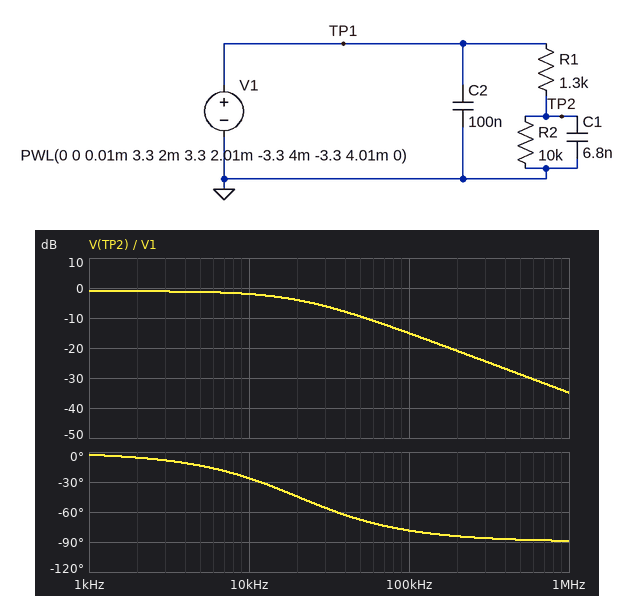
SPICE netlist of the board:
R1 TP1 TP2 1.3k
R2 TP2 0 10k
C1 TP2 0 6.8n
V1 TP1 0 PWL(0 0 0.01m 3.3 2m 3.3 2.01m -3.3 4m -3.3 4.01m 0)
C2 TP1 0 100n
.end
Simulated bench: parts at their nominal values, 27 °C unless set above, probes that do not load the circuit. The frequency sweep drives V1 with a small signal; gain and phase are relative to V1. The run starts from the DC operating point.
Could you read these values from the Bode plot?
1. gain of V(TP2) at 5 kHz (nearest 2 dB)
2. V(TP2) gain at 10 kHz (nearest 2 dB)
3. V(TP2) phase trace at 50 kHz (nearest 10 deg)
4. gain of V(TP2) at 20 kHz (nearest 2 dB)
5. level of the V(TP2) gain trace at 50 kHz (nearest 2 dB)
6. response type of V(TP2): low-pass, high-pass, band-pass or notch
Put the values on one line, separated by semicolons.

-2 dB; -2 dB; -70 deg; -4 dB; -10 dB; low-pass
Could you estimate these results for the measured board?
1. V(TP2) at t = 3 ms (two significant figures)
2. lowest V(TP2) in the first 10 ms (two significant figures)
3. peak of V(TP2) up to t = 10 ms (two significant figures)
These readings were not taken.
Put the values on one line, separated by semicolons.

-2.9 V; -2.9 V; 2.9 V
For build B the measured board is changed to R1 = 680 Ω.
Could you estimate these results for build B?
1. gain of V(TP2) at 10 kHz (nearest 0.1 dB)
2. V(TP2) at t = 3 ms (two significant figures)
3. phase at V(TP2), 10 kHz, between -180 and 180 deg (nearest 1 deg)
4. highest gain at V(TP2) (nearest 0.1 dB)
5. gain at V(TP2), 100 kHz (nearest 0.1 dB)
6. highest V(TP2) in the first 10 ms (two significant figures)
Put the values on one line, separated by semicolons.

-0.9 dB; -3.1 V; -15 deg; -0.6 dB; -9.8 dB; 3.1 V
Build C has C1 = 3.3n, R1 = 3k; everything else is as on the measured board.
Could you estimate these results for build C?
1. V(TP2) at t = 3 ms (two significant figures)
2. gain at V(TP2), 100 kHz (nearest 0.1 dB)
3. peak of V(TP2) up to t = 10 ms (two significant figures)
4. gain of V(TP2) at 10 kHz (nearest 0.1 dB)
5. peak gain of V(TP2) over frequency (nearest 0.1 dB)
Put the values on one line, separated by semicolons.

-2.5 V; -16.1 dB; 2.5 V; -3.2 dB; -2.3 dB
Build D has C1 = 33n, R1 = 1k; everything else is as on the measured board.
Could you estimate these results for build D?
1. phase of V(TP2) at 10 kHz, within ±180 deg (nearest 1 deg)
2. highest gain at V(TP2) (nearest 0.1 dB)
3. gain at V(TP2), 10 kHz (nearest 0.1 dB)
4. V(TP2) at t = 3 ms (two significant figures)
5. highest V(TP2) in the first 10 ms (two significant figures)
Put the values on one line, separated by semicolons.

-62 deg; -0.8 dB; -7.4 dB; -3.0 V; 3.0 V
